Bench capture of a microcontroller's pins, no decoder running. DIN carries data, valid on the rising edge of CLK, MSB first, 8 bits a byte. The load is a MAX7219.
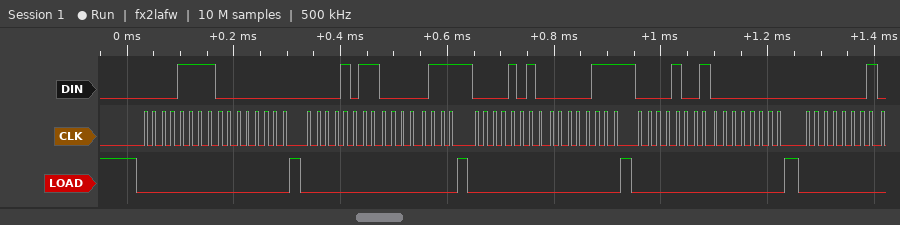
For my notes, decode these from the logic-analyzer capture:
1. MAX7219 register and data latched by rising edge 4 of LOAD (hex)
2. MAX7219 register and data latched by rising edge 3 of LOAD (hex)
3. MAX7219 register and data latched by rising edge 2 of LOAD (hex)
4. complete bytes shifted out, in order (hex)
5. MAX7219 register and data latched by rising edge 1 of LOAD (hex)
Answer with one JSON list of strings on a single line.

["register 0x9, data 0x00", "register 0xA, data 0x07", "register 0xB, data 0x07", "0x0F 0x00 0x0B 0x07 0x0A 0x07 0x09 0x00 0x01", "register 0xF, data 0x00"]
